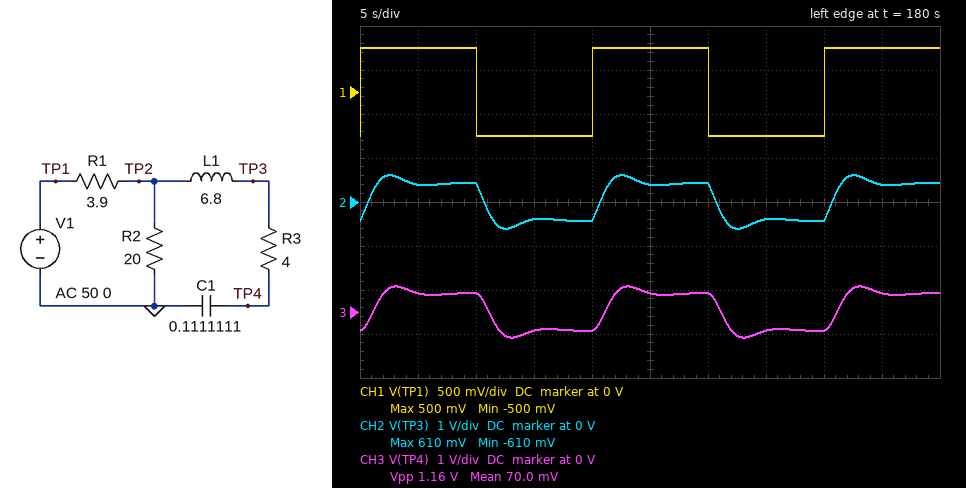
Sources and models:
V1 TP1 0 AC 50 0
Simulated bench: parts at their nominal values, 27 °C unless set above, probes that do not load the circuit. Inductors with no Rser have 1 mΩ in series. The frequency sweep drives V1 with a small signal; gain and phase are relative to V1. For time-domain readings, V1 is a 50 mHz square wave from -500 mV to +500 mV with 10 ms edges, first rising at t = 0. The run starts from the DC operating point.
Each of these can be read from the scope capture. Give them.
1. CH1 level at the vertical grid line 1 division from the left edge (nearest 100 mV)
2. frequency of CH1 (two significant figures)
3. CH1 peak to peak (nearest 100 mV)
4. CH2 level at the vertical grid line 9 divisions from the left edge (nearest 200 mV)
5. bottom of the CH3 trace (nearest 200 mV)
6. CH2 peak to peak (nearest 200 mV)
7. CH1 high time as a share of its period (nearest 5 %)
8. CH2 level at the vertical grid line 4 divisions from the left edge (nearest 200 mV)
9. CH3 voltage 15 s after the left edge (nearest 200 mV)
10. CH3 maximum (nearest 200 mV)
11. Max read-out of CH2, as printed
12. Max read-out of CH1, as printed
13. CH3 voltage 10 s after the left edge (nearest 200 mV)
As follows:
500 mV
50 mHz
1.0 V
400 mV
-600 mV
1.2 V
50 %
-400 mV
-400 mV
600 mV
610 mV
500 mV
400 mV
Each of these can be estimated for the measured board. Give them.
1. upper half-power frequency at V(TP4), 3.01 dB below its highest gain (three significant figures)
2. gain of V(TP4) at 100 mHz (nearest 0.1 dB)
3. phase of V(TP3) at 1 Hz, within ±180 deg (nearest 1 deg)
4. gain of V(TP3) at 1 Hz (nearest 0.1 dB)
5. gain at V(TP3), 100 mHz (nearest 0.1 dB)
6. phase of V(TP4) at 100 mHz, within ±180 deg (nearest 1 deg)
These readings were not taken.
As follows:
216 mHz
-0.3 dB
-100 deg
-21.4 dB
0 dB
-36 deg
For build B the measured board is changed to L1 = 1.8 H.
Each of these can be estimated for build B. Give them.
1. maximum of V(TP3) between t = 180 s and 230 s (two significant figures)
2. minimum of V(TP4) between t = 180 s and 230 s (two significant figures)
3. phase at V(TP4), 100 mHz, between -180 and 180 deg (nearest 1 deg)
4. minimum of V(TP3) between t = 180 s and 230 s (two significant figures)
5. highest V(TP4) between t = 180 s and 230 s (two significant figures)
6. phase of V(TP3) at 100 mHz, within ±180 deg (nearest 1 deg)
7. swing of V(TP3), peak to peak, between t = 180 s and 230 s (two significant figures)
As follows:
430 mV
-420 mV
-29 deg
-430 mV
420 mV
-13 deg
850 mV
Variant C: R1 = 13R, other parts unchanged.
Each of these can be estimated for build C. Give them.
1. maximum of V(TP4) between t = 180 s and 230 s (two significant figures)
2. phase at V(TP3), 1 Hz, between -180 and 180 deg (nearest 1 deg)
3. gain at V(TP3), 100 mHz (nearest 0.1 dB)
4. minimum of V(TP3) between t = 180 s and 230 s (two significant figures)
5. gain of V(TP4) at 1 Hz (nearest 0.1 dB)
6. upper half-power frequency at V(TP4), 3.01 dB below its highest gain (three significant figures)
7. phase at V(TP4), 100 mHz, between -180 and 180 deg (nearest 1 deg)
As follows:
320 mV
-94 deg
-4.7 dB
-320 mV
-33.9 dB
170 mHz
-50 deg
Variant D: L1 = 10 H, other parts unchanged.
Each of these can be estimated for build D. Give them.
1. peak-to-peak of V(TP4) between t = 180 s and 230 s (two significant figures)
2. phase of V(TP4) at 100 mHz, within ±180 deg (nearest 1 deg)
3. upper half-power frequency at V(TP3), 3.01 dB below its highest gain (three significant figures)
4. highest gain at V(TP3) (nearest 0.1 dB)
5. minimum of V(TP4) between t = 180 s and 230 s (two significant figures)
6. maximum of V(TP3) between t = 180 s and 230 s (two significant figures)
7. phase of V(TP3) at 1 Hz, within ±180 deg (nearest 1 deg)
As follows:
1.3 V
-42 deg
185 mHz
2.0 dB
-650 mV
670 mV
-103 deg
